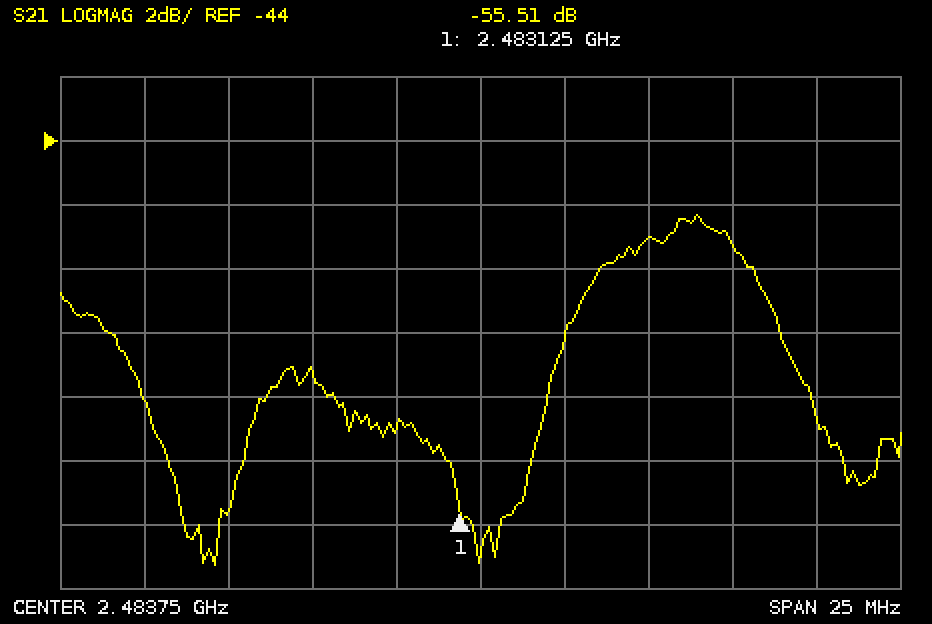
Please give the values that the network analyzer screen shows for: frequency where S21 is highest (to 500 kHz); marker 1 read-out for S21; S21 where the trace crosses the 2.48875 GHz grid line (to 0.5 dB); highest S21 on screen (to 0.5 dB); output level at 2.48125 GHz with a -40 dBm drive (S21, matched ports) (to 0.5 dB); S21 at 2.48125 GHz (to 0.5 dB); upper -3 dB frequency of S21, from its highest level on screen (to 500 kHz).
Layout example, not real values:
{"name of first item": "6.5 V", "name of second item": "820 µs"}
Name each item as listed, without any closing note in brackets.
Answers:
{"frequency where S21 is highest": "2.4900 GHz", "marker 1 read-out for S21": "-55.51 dB", "S21 where the trace crosses the 2.48875 GHz grid line": "-47.0 dB", "highest S21 on screen": "-46.5 dB", "output level at 2.48125 GHz with a -40 dBm drive (S21, matched ports)": "-93.0 dBm", "S21 at 2.48125 GHz": "-53.0 dB", "upper -3 dB frequency of S21, from its highest level on screen": "2.4925 GHz"}
